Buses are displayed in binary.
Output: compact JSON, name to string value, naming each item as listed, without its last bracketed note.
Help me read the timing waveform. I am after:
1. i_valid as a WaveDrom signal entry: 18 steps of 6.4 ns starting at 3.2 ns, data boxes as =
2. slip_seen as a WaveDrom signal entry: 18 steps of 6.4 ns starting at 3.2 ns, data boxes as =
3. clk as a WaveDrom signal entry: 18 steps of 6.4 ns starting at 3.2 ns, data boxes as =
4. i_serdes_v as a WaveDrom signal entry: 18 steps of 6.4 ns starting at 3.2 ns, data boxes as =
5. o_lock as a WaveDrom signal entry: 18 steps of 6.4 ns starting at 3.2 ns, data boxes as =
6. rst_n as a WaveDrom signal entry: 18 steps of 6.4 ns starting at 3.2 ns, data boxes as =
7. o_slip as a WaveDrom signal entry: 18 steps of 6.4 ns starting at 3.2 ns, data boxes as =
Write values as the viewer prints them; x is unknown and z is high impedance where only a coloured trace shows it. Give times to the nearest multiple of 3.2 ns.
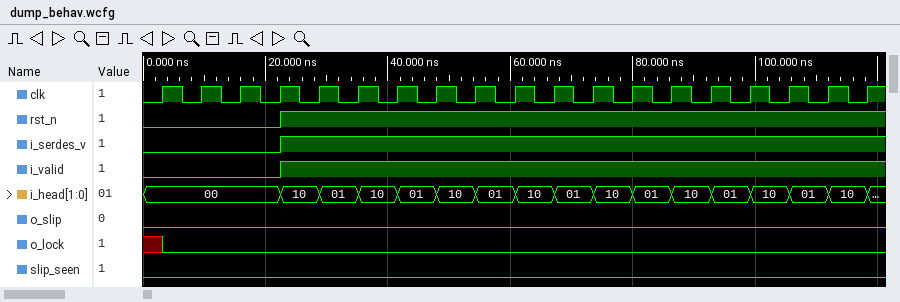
{"i_valid as a WaveDrom signal entry: 18 steps of 6.4 ns starting at 3.2 ns, data boxes as =": "{name: 'i_valid', wave: '0..1..............'}", "slip_seen as a WaveDrom signal entry: 18 steps of 6.4 ns starting at 3.2 ns, data boxes as =": "{name: 'slip_seen', wave: '0.................'}", "clk as a WaveDrom signal entry: 18 steps of 6.4 ns starting at 3.2 ns, data boxes as =": "{name: 'clk', wave: 'p.................'}", "i_serdes_v as a WaveDrom signal entry: 18 steps of 6.4 ns starting at 3.2 ns, data boxes as =": "{name: 'i_serdes_v', wave: '0..1..............'}", "o_lock as a WaveDrom signal entry: 18 steps of 6.4 ns starting at 3.2 ns, data boxes as =": "{name: 'o_lock', wave: '0.................'}", "rst_n as a WaveDrom signal entry: 18 steps of 6.4 ns starting at 3.2 ns, data boxes as =": "{name: 'rst_n', wave: '0..1..............'}", "o_slip as a WaveDrom signal entry: 18 steps of 6.4 ns starting at 3.2 ns, data boxes as =": "{name: 'o_slip', wave: '0.................'}"}
